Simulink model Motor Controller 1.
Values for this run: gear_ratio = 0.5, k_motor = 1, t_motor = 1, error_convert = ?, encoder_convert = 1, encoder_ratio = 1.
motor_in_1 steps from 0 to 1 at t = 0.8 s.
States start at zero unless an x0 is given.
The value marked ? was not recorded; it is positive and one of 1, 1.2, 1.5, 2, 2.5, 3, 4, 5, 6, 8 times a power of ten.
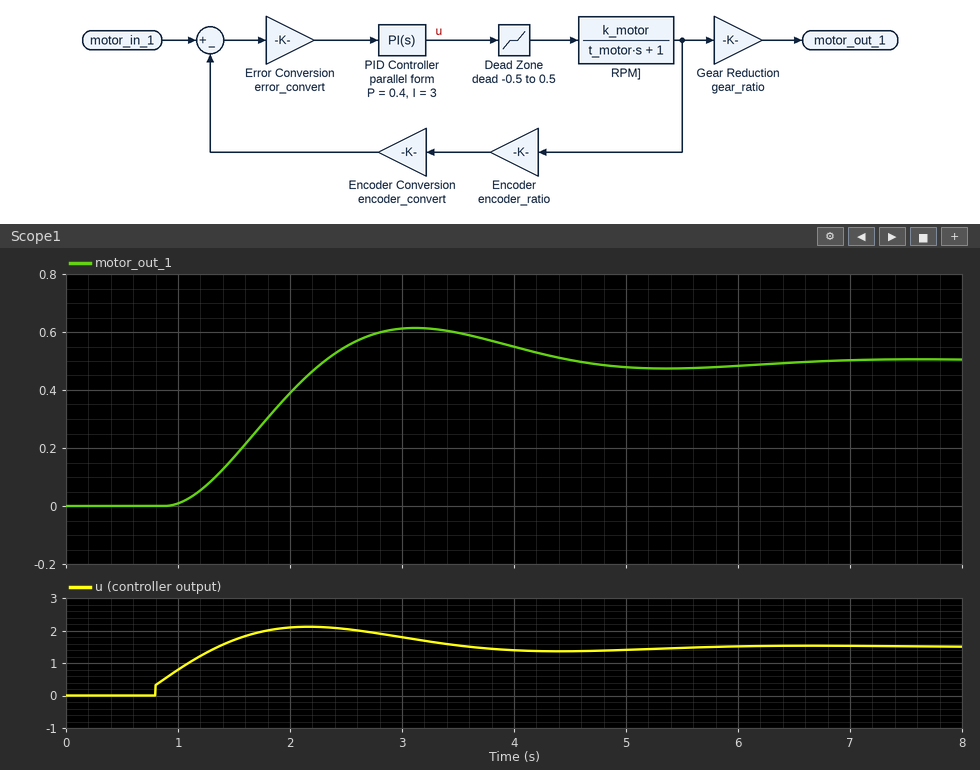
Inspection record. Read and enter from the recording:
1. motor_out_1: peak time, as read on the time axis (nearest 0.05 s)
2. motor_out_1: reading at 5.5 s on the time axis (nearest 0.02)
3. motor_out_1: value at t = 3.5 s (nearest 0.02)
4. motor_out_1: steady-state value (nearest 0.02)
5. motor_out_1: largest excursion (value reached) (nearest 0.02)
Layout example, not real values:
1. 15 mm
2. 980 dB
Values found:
1. 3.10 s
2. 0.48
3. 0.60
4. 0.50
5. 0.62
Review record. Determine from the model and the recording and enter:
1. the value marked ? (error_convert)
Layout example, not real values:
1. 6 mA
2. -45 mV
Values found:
1. 0.8
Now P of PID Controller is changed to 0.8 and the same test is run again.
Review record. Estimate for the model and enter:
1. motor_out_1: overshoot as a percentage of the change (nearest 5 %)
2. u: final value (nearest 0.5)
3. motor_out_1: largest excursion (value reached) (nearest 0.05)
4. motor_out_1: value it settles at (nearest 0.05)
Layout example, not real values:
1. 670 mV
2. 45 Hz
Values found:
1. 15 %
2. 1.5
3. 0.55
4. 0.50
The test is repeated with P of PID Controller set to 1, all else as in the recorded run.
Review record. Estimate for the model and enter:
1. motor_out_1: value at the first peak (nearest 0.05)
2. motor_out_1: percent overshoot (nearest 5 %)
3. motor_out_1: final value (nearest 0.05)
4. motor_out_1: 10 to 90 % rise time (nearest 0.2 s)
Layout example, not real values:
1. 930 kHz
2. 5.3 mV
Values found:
1. 0.55
2. 10 %
3. 0.50
4. 1.2 s
